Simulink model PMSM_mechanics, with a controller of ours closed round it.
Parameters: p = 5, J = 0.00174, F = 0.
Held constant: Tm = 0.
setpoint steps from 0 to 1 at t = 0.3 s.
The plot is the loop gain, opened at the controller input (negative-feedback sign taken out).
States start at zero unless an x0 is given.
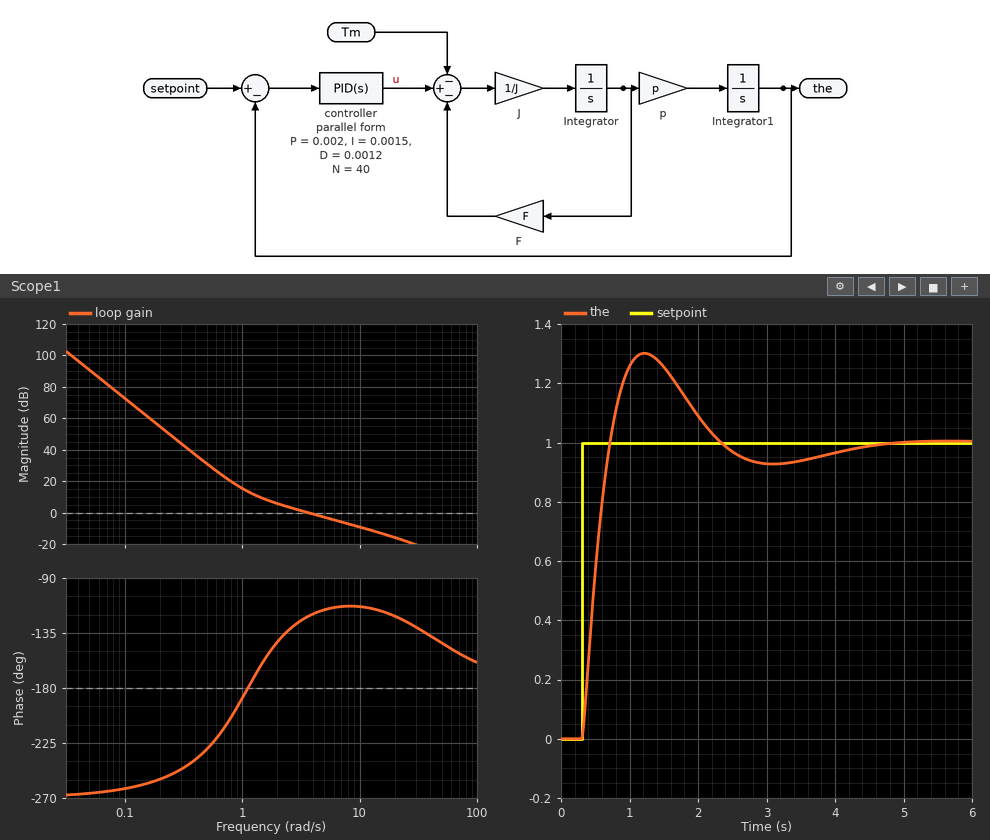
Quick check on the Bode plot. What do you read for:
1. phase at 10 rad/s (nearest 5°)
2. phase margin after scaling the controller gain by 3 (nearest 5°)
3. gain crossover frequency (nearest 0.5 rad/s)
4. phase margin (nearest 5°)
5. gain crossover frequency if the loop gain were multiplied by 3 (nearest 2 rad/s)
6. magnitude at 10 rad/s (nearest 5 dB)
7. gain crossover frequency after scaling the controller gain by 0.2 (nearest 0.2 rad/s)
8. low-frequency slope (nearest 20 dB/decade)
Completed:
-115°
65°
3.5 rad/s
60°
10 rad/s
-10 dB
1.0 rad/s
-60 dB/decade
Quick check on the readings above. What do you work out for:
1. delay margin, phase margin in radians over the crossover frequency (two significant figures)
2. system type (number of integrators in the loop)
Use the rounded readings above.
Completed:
0.30 s
3
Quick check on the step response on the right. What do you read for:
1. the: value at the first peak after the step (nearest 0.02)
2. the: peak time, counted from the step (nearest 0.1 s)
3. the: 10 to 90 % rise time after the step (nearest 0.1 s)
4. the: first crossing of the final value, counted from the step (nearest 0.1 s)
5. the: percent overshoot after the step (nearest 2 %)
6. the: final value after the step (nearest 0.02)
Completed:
1.30
0.9 s
0.3 s
0.4 s
30 %
1.00
